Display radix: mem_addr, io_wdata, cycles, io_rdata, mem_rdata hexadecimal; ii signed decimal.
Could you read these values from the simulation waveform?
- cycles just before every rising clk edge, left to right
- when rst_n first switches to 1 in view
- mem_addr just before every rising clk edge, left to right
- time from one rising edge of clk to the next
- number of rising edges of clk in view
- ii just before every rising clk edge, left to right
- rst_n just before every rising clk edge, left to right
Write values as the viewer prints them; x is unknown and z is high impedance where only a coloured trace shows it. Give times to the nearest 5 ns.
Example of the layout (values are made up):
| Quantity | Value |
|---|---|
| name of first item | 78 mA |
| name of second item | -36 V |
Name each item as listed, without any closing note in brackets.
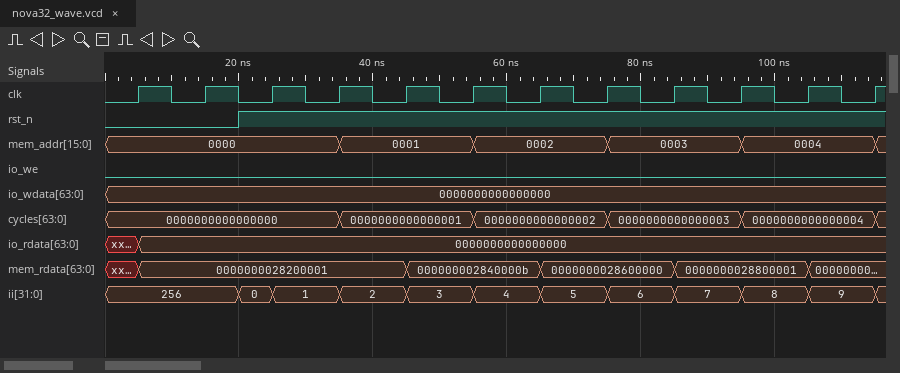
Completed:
| Quantity | Value |
|---|---|
| cycles just before every rising clk edge, left to right | 0000000000000000, 0000000000000000, 0000000000000000, 0000000000000000, 0000000000000001, 0000000000000001, 0000000000000002, 0000000000000002, 0000000000000003, 0000000000000003, 0000000000000004, 0000000000000004 |
| when rst_n first switches to 1 in view | 20 ns |
| mem_addr just before every rising clk edge, left to right | 0000, 0000, 0000, 0000, 0001, 0001, 0002, 0002, 0003, 0003, 0004, 0004 |
| time from one rising edge of clk to the next | 10 ns |
| number of rising edges of clk in view | 12 |
| ii just before every rising clk edge, left to right | 256, 256, 0, 1, 2, 3, 4, 5, 6, 7, 8, 9 |
| rst_n just before every rising clk edge, left to right | 0 0 1 1 1 1 1 1 1 1 1 1 |
